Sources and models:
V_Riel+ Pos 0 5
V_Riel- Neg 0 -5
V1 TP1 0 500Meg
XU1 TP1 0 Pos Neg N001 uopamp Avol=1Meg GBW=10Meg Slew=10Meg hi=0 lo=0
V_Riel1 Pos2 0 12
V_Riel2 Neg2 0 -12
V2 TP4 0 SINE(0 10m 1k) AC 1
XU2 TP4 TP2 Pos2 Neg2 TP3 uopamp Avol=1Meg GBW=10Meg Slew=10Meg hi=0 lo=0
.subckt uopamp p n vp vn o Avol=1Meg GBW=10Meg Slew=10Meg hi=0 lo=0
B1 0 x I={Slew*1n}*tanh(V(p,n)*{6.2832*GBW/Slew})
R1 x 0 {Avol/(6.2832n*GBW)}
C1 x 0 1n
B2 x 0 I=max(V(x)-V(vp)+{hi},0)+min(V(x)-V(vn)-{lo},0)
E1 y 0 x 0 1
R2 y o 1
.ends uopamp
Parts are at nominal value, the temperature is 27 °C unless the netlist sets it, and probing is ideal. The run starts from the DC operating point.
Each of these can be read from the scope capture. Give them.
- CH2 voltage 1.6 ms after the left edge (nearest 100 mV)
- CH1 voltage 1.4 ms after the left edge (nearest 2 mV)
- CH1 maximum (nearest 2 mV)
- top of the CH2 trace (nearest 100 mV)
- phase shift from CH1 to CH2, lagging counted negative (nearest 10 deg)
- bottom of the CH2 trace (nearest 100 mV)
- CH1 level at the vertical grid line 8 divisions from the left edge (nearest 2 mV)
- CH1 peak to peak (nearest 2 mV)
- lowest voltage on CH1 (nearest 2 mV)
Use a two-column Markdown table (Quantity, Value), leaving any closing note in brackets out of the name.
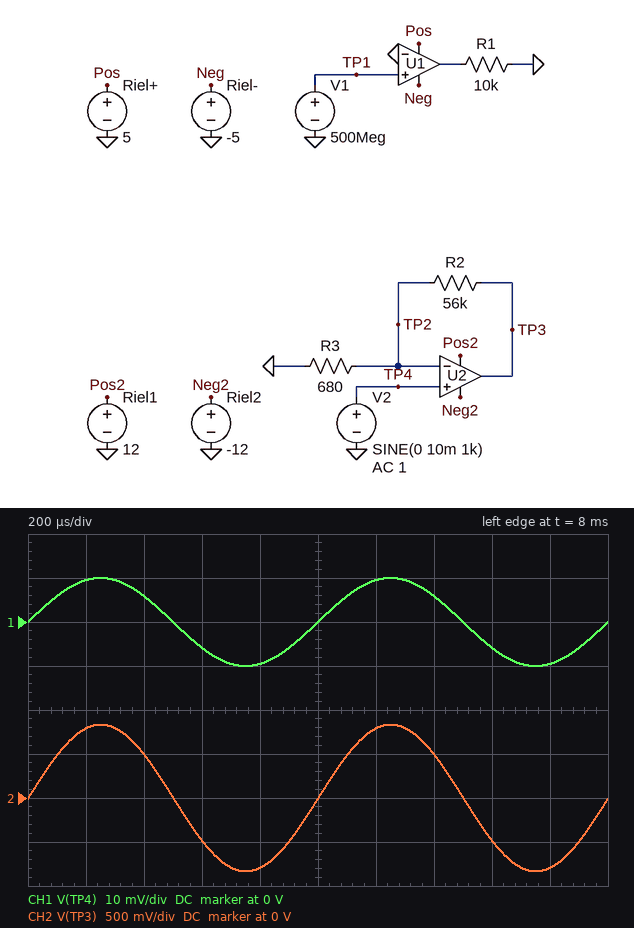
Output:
| Quantity | Value |
|---|---|
| CH2 voltage 1.6 ms after the left edge | -500 mV |
| CH1 voltage 1.4 ms after the left edge | 6 mV |
| CH1 maximum | 10 mV |
| top of the CH2 trace | 800 mV |
| phase shift from CH1 to CH2, lagging counted negative | 0 deg |
| bottom of the CH2 trace | -800 mV |
| CH1 level at the vertical grid line 8 divisions from the left edge | -6 mV |
| CH1 peak to peak | 20 mV |
| lowest voltage on CH1 | -10 mV |
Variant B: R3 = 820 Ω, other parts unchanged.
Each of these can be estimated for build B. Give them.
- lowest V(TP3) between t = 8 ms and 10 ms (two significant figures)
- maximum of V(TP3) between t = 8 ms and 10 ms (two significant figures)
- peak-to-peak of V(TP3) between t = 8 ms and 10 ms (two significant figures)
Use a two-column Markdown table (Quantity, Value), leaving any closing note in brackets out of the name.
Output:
| Quantity | Value |
|---|---|
| lowest V(TP3) between t = 8 ms and 10 ms | -690 mV |
| maximum of V(TP3) between t = 8 ms and 10 ms | 690 mV |
| peak-to-peak of V(TP3) between t = 8 ms and 10 ms | 1.4 V |
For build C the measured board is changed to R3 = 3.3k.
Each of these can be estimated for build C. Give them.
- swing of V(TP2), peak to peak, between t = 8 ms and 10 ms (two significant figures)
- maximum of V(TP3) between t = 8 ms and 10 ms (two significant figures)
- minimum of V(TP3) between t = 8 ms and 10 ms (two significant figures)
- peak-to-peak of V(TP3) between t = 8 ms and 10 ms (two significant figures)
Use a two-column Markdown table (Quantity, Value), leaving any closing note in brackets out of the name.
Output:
| Quantity | Value |
|---|---|
| swing of V(TP2), peak to peak, between t = 8 ms and 10 ms | 20 mV |
| maximum of V(TP3) between t = 8 ms and 10 ms | 180 mV |
| minimum of V(TP3) between t = 8 ms and 10 ms | -180 mV |
| peak-to-peak of V(TP3) between t = 8 ms and 10 ms | 360 mV |
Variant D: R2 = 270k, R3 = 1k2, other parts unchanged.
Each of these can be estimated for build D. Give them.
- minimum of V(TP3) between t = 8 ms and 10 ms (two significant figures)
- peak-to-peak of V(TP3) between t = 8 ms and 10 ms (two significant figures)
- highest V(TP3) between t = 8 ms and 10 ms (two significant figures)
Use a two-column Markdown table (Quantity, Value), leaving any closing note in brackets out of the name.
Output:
| Quantity | Value |
|---|---|
| minimum of V(TP3) between t = 8 ms and 10 ms | -2.3 V |
| peak-to-peak of V(TP3) between t = 8 ms and 10 ms | 4.5 V |
| highest V(TP3) between t = 8 ms and 10 ms | 2.3 V |
